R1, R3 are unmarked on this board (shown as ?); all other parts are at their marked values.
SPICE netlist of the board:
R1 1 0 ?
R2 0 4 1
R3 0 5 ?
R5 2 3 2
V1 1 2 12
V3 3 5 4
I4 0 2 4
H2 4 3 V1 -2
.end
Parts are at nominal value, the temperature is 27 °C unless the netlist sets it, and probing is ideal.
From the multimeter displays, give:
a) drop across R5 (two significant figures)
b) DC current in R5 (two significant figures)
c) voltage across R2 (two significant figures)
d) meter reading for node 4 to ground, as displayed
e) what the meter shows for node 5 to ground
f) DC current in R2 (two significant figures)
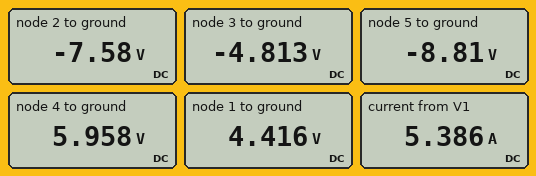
2.8 V
1.4 A
6.0 V
5.958 V
-8.81 V
6.0 A
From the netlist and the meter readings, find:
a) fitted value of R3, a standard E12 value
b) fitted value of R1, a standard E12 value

1.2 Ω
0.82 Ω
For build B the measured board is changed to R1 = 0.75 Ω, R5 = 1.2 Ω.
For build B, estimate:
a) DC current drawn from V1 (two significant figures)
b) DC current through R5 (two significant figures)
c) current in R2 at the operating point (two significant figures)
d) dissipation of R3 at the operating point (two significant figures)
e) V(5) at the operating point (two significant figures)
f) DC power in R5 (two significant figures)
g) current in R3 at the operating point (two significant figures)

5.8 A
1.8 A
6.1 A
75 W
-9.5 V
3.9 W
7.9 A
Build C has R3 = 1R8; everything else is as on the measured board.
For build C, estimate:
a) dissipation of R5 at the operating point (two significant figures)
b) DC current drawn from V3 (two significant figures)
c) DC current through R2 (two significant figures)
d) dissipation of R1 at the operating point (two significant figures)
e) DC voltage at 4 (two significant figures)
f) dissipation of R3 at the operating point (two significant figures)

2.2 W
5.4 A
4.4 A
21 W
4.4 V
53 W
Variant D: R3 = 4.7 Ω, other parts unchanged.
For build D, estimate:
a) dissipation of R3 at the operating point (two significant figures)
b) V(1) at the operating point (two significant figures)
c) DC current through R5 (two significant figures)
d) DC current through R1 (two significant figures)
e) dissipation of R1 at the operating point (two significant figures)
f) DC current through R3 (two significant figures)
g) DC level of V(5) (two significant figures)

27 W
3.7 V
530 mA
4.5 A
17 W
2.4 A
-11 V
